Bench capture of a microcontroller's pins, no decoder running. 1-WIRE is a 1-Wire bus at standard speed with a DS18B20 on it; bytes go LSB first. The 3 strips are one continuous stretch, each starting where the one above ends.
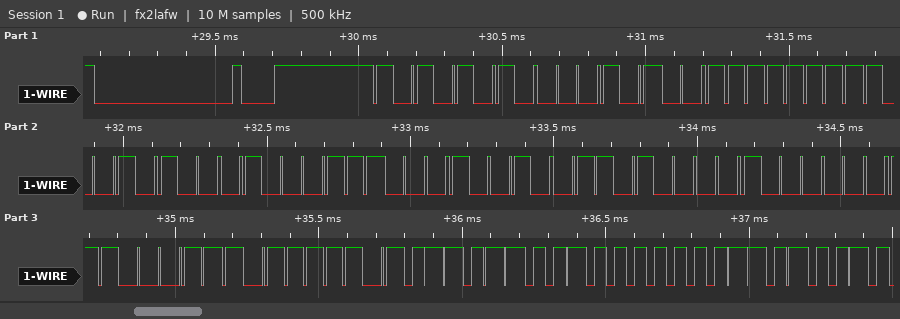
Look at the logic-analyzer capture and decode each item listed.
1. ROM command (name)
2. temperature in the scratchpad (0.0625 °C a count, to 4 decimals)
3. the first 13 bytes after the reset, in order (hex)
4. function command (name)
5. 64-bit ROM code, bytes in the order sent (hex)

Match ROM
19.3750 °C
55 28 FF 29 E2 48 16 02 E3 BE 36 01 4B
Read Scratchpad
28 FF 29 E2 48 16 02 E3
